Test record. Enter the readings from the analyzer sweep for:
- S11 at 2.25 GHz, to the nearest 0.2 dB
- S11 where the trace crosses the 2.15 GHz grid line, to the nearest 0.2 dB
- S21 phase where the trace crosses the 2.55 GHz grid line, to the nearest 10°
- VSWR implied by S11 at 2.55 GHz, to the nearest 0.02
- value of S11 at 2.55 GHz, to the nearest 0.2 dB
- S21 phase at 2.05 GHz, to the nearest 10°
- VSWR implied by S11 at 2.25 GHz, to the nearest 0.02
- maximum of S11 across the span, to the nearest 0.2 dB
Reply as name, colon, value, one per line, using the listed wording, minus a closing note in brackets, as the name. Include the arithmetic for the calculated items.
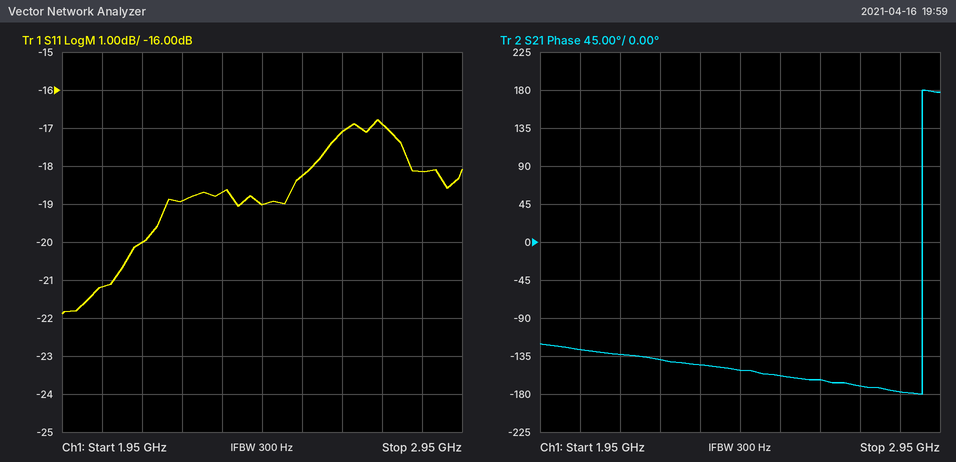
S11 at 2.25 GHz, to the nearest 0.2 dB: -19.0 dB
S11 where the trace crosses the 2.15 GHz grid line, to the nearest 0.2 dB: -20.0 dB
S21 phase where the trace crosses the 2.55 GHz grid line, to the nearest 10°: -160°
VSWR implied by S11 at 2.55 GHz, to the nearest 0.02: |Γ| = 10^(-18.2/20) = 0.1230; VSWR = (1 + 0.1230)/(1 − 0.1230) ≈ 1.28
value of S11 at 2.55 GHz, to the nearest 0.2 dB: -18.2 dB
S21 phase at 2.05 GHz, to the nearest 10°: -130°
VSWR implied by S11 at 2.25 GHz, to the nearest 0.02: |Γ| = 10^(-19/20) = 0.1122; VSWR = (1 + 0.1122)/(1 − 0.1122) ≈ 1.25, so 1.26 to the nearest 0.02
maximum of S11 across the span, to the nearest 0.2 dB: -16.8 dB
